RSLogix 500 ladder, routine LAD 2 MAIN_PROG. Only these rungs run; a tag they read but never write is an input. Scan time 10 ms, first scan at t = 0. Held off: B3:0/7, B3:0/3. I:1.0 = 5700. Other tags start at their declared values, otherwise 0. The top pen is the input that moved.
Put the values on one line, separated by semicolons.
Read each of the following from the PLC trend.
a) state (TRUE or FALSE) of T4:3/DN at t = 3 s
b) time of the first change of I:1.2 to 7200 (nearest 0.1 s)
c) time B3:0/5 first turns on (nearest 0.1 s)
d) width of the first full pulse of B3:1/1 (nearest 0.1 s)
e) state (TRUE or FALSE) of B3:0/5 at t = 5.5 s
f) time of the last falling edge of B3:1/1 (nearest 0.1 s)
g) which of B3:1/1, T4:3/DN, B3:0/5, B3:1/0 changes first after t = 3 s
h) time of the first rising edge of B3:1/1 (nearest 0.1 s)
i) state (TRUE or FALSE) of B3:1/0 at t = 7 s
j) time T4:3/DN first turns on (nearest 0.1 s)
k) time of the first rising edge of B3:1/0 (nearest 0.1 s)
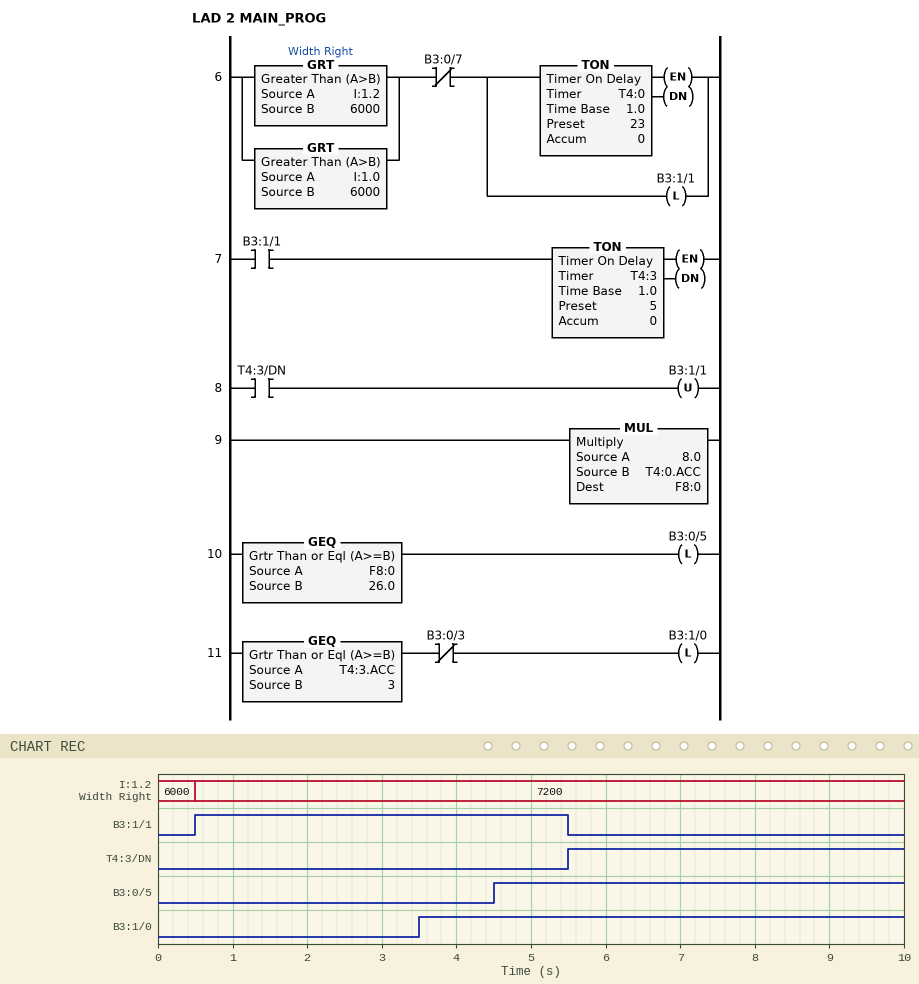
FALSE; 0.5 s; 4.5 s; 5.0 s; TRUE; 5.5 s; B3:1/0; 0.5 s; TRUE; 5.5 s; 3.5 s
